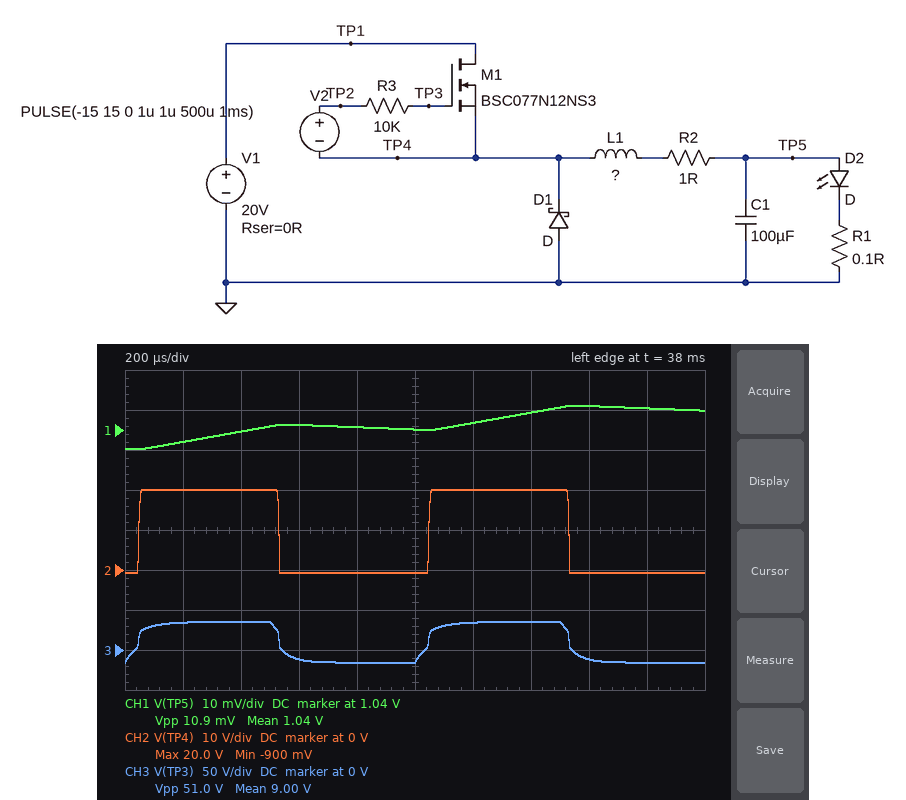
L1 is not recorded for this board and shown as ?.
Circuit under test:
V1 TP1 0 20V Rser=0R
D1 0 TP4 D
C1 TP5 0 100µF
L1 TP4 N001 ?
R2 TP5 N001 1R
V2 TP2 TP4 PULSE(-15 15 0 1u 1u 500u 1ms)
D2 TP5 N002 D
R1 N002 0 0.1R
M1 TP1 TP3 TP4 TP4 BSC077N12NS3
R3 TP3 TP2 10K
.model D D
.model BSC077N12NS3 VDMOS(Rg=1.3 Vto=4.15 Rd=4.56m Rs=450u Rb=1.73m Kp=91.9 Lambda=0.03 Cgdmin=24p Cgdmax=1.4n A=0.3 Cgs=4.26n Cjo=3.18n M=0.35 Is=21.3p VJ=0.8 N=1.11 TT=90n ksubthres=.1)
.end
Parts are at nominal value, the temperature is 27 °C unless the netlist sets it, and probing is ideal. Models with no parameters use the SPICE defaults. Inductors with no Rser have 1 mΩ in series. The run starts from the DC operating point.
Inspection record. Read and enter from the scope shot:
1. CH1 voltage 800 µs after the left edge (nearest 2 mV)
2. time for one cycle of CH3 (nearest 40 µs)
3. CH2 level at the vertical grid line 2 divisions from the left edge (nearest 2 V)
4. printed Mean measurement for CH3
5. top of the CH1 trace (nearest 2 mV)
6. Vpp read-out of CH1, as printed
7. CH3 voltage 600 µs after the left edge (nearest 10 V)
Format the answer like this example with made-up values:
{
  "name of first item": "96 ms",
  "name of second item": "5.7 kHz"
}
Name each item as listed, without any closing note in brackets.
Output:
{
  "CH1 voltage 800 µs after the left edge": "1.040 V",
  "time for one cycle of CH3": "1.00 ms",
  "CH2 level at the vertical grid line 2 divisions from the left edge": "20 V",
  "printed Mean measurement for CH3": "9.00 V",
  "top of the CH1 trace": "1.046 V",
  "Vpp read-out of CH1, as printed": "10.9 mV",
  "CH3 voltage 600 µs after the left edge": "-10 V"
}
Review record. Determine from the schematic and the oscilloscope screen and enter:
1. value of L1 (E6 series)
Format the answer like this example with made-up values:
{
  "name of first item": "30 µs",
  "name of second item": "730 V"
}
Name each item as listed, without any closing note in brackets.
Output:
{
  "value of L1": "150 mH"
}
